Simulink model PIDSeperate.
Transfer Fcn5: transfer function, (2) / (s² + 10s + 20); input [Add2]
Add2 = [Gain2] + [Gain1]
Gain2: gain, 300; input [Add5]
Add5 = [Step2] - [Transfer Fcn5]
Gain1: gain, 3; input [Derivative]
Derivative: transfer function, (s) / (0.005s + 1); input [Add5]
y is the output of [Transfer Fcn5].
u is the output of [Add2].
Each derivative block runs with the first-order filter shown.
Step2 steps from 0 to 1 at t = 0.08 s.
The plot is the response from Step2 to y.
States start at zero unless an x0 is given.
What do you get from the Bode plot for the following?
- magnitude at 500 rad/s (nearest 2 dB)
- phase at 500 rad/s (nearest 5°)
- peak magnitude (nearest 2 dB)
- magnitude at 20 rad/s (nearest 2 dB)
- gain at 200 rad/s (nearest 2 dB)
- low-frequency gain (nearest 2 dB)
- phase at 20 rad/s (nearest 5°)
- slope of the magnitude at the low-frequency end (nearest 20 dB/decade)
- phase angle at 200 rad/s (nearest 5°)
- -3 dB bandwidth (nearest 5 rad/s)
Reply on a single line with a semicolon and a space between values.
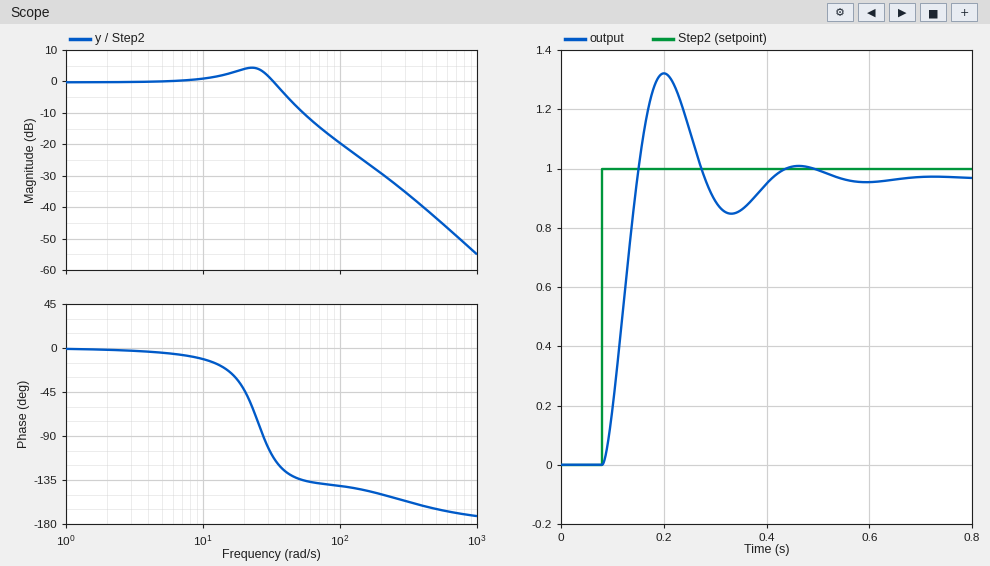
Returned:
-44 dB; -165°; 4 dB; 4 dB; -30 dB; 0 dB; -45°; 0 dB/decade; -150°; 40 rad/s
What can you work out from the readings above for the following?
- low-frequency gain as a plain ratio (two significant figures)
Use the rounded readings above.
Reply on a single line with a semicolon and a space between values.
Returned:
1.0
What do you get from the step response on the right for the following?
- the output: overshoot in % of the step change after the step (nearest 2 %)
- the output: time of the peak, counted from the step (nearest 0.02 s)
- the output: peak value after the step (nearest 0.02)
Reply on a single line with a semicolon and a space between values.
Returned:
36 %; 0.12 s; 1.32
